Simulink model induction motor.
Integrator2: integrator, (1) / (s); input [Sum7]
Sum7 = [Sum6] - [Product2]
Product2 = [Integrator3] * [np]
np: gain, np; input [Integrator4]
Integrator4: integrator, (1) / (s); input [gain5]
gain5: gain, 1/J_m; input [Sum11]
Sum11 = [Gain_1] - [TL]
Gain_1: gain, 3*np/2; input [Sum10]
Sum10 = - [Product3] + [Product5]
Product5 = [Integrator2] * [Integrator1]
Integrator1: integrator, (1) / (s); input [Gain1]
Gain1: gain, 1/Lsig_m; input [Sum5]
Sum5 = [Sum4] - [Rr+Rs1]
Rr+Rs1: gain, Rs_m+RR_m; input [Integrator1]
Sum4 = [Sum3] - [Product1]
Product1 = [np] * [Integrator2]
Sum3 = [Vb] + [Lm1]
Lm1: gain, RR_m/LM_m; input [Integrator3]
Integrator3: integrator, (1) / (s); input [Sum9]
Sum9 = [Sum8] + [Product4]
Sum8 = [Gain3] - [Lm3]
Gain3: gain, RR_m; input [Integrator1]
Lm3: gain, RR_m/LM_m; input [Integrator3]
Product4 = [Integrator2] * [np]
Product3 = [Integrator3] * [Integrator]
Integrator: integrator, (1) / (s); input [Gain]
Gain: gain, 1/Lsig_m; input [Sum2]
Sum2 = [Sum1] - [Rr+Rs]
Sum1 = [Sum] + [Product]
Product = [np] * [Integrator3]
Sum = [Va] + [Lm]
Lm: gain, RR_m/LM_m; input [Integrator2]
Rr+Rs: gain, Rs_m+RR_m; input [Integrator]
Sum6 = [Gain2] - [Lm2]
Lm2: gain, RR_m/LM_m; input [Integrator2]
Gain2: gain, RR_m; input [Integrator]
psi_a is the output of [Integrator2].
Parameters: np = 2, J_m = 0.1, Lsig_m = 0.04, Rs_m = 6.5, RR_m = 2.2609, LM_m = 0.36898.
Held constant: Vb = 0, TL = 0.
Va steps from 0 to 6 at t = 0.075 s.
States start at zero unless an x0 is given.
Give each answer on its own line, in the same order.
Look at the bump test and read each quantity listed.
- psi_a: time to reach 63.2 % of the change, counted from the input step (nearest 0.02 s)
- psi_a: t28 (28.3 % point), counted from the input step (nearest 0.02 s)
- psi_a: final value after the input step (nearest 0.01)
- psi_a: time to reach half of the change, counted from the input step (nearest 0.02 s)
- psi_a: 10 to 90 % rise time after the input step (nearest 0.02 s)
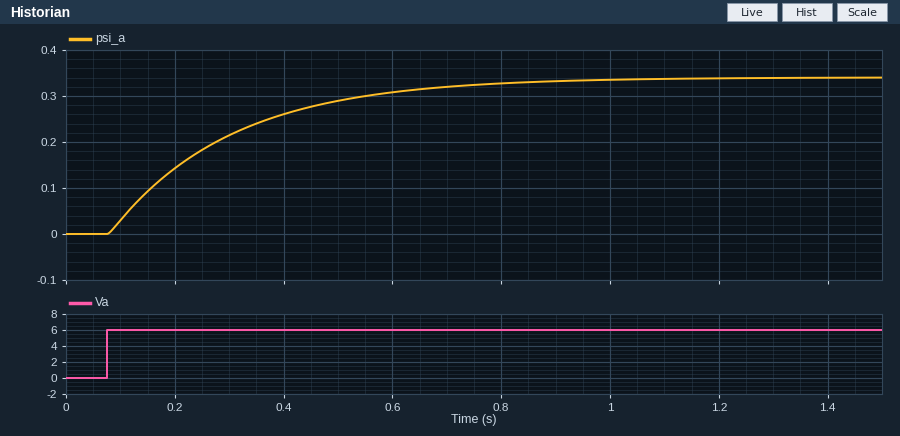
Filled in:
0.22 s
0.08 s
0.34
0.16 s
0.48 s
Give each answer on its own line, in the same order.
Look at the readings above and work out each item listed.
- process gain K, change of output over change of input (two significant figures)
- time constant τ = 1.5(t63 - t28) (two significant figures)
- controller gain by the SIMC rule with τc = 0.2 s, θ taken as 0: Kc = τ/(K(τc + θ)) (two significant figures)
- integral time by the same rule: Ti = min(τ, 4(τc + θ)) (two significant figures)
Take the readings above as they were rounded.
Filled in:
0.057
0.21 s
18
0.21 s
